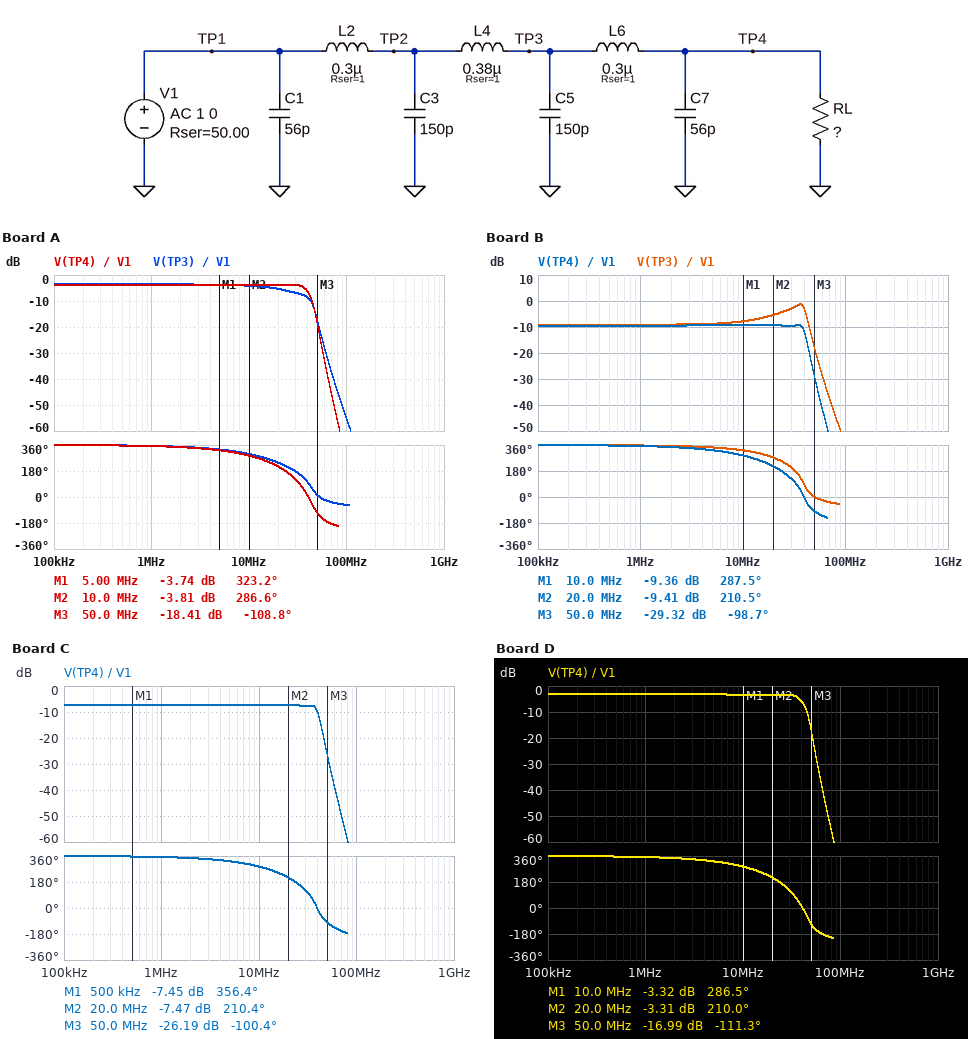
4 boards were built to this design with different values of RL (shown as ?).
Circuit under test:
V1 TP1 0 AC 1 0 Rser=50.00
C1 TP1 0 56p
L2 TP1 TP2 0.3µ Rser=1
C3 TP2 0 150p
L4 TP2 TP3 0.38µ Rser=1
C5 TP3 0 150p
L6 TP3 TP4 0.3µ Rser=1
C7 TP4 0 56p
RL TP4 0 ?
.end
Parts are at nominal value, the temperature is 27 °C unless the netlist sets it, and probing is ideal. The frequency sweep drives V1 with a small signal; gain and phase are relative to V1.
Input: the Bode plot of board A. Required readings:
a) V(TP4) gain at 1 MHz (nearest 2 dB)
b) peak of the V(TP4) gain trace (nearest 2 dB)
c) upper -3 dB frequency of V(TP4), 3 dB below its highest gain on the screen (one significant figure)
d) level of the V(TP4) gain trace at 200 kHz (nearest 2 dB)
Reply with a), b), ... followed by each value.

a) -4 dB
b) -4 dB
c) 40 MHz
d) -4 dB
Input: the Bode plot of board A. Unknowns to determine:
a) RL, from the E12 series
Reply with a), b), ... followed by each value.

a) 100 Ω
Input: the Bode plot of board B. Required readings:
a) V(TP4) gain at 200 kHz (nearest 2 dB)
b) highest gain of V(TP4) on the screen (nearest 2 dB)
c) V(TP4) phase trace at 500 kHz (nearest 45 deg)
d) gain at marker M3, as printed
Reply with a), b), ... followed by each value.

a) -10 dB
b) -10 dB
c) 360 deg
d) -29.32 dB
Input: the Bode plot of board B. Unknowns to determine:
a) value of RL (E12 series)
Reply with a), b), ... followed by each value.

a) 27 Ω
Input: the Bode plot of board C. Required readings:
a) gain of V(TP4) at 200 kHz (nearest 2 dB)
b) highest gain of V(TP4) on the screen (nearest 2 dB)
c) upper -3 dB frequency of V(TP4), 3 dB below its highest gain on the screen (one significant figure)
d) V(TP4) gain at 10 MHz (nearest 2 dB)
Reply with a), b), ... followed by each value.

a) -8 dB
b) -8 dB
c) 40 MHz
d) -8 dB
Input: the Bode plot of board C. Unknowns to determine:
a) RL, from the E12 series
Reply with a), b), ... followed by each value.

a) 39 Ω
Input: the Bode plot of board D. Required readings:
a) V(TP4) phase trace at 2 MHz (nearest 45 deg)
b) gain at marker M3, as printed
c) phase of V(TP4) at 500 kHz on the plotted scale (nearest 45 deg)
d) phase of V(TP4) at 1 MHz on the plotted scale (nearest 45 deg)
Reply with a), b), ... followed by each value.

a) 360 deg
b) -16.99 dB
c) 360 deg
d) 360 deg
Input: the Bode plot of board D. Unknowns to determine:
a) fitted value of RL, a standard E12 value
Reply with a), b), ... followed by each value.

a) 120 Ω
